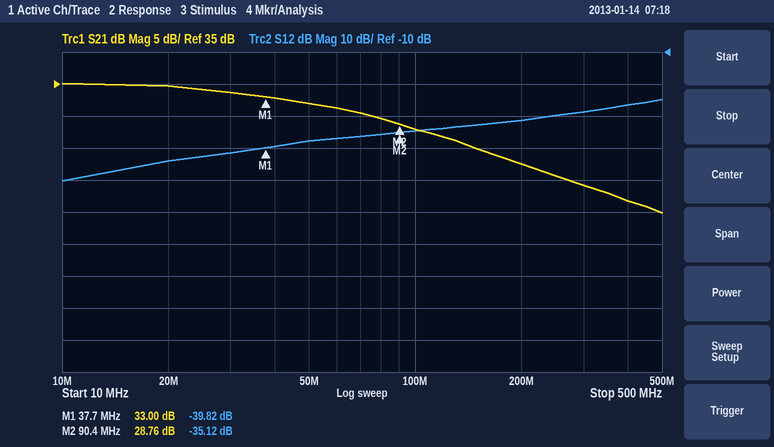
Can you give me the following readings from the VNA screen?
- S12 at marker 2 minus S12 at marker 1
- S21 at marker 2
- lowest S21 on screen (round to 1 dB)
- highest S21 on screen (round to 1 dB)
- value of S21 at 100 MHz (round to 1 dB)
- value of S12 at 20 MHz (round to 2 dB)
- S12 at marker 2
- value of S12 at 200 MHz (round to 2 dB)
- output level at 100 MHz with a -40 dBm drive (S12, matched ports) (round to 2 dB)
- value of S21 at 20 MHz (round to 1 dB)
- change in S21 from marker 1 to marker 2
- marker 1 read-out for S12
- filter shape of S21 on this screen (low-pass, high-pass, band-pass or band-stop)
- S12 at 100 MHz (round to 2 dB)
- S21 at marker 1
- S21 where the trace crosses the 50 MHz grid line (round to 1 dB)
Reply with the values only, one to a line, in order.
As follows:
4.70 dB
28.76 dB
15 dB
35 dB
28 dB
-44 dB
-35.12 dB
-32 dB
-74 dBm
35 dB
-4.24 dB
-39.82 dB
low-pass
-34 dB
33.00 dB
32 dB
